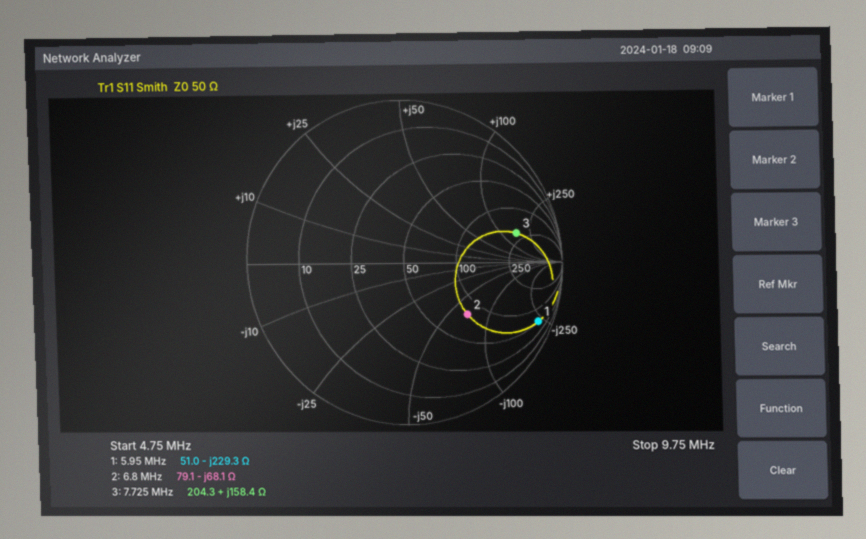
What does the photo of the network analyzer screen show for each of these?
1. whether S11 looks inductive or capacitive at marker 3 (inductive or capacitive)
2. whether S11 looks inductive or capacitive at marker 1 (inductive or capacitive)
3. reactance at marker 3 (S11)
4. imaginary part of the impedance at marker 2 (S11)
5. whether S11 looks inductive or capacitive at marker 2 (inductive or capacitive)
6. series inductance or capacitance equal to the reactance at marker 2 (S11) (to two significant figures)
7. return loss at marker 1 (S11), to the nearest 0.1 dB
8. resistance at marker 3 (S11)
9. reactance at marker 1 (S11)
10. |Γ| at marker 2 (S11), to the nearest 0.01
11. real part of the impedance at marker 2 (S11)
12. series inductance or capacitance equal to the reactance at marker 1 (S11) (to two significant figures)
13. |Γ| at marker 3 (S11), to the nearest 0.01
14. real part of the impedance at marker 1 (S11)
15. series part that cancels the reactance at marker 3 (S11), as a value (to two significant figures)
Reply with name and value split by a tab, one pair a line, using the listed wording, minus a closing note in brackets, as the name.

whether S11 looks inductive or capacitive at marker 3	inductive
whether S11 looks inductive or capacitive at marker 1	capacitive
reactance at marker 3	+158.4 Ω
imaginary part of the impedance at marker 2	-68.1 Ω
whether S11 looks inductive or capacitive at marker 2	capacitive
series inductance or capacitance equal to the reactance at marker 2 (S11)	340 pF
return loss at marker 1 (S11), to the nearest 0.1 dB	0.8 dB
resistance at marker 3	204.3 Ω
reactance at marker 1	-229.3 Ω
|Γ| at marker 2 (S11), to the nearest 0.01	0.51
real part of the impedance at marker 2	79.1 Ω
series inductance or capacitance equal to the reactance at marker 1 (S11)	120 pF
|Γ| at marker 3 (S11), to the nearest 0.01	0.74
real part of the impedance at marker 1	51.0 Ω
series part that cancels the reactance at marker 3 (S11), as a value	130 pF
